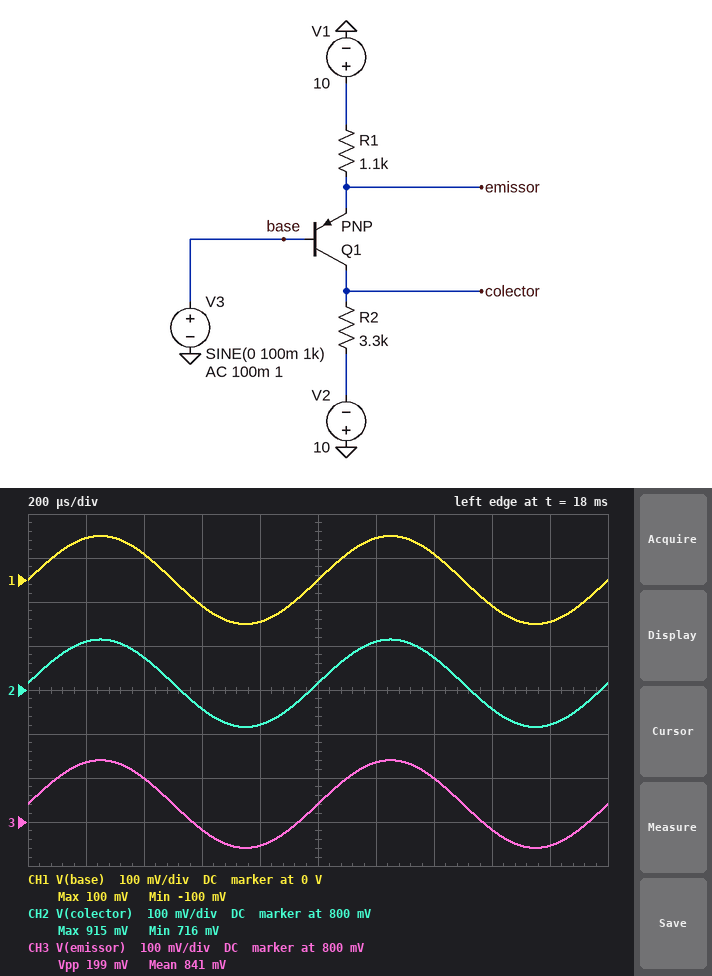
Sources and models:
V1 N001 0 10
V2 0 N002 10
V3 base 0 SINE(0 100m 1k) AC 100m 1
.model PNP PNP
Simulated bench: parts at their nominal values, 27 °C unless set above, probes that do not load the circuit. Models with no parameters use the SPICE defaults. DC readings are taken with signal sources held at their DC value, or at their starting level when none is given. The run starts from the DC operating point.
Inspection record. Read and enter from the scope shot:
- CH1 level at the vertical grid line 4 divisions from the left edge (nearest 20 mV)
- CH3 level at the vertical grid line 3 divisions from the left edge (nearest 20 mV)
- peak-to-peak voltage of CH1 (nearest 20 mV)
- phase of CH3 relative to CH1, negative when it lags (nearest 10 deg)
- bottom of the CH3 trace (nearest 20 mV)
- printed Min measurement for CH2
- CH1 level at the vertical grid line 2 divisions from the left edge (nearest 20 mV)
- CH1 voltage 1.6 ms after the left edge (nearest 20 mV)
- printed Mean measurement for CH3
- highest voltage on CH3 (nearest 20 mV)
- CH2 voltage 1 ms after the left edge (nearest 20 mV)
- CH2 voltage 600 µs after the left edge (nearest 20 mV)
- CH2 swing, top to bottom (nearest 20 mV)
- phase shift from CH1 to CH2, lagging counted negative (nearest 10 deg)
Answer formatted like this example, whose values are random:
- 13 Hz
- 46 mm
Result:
- -100 mV
- 780 mV
- 200 mV
- 0 deg
- 740 mV
- 716 mV
- 60 mV
- -60 mV
- 841 mV
- 940 mV
- 820 mV
- 760 mV
- 200 mV
- 0 deg
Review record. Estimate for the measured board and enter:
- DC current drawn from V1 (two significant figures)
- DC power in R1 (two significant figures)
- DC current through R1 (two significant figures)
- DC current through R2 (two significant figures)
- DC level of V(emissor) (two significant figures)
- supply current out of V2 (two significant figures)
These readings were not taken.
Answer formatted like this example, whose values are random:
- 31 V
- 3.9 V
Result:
- 8.3 mA
- 76 mW
- 8.3 mA
- 3.3 mA
- 840 mV
- 3.3 mA
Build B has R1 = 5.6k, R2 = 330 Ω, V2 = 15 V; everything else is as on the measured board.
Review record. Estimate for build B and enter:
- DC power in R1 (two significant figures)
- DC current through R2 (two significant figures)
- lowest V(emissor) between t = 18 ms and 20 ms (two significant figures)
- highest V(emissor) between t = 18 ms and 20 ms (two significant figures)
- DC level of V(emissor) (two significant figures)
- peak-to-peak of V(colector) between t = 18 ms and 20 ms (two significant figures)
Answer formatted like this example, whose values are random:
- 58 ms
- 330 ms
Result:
- 15 mW
- 1.6 mA
- 690 mV
- 890 mV
- 790 mV
- 12 mV
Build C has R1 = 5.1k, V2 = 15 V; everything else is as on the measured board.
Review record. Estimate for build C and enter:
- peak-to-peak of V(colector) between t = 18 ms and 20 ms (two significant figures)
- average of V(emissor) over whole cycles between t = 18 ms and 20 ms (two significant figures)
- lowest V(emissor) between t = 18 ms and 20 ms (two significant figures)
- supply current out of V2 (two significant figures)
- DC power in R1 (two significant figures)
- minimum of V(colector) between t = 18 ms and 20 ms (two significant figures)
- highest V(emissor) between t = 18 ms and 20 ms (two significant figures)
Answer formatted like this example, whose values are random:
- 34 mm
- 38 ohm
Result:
- 130 mV
- 790 mV
- 690 mV
- 1.8 mA
- 17 mW
- -9.2 V
- 890 mV
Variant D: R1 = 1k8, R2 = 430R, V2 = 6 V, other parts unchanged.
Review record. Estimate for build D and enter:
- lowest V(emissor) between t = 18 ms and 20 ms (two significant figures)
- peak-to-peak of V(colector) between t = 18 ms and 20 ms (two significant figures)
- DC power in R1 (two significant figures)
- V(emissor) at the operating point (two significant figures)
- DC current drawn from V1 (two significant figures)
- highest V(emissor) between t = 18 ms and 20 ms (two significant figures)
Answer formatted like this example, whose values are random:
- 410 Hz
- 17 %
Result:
- 720 mV
- 47 mV
- 47 mW
- 820 mV
- 5.1 mA
- 920 mV
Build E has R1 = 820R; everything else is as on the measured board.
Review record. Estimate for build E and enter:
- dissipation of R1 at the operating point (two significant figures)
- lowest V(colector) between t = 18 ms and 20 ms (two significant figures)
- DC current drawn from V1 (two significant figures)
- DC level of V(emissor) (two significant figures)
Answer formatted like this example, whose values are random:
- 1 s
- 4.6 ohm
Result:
- 100 mW
- 730 mV
- 11 mA
- 850 mV
